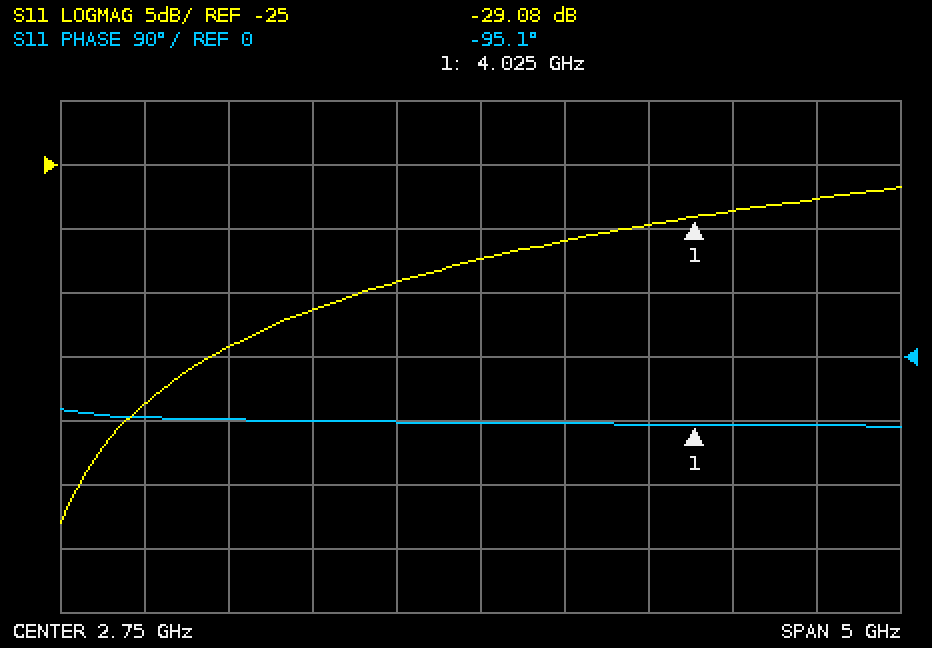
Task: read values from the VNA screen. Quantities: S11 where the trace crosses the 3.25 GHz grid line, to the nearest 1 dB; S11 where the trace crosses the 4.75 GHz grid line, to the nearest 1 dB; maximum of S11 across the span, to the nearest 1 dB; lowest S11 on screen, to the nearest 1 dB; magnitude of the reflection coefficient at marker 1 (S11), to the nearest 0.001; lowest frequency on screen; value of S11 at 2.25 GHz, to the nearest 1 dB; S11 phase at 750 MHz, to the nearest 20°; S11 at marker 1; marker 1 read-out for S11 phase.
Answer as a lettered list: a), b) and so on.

a) -31 dB
b) -28 dB
c) -27 dB
d) -53 dB
e) 0.035
f) 250 MHz
g) -34 dB
h) -80°
i) -29.08 dB
j) -95.1°
